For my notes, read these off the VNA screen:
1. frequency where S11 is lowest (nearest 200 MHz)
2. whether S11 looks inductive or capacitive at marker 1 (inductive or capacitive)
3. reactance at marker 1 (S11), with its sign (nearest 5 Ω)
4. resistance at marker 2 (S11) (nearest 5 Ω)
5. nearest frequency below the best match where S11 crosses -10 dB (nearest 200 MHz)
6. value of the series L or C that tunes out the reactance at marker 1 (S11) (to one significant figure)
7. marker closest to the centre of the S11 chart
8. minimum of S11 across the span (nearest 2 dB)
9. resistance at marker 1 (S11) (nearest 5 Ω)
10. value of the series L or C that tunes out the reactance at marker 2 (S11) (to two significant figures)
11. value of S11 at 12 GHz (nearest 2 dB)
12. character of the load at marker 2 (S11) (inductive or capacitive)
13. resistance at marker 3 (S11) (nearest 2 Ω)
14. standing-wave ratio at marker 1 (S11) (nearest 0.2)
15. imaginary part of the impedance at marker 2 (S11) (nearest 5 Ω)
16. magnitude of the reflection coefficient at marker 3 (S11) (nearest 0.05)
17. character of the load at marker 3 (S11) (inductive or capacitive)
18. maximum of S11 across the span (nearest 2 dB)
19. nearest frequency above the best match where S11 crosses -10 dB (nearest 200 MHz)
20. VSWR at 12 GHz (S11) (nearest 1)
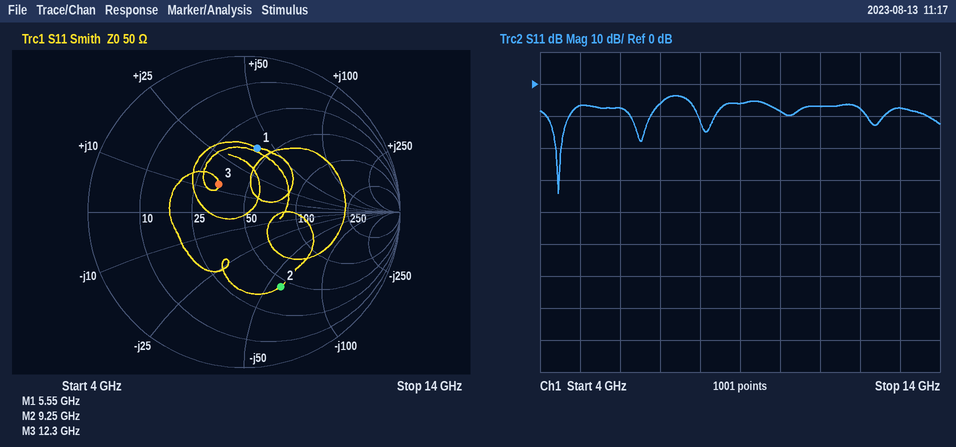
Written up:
4.4 GHz
inductive
+40 Ω
45 Ω
4.2 GHz
700 fF
marker 3
-34 dB
40 Ω
1.0 nH
-8 dB
capacitive
34 Ω
2.4
-60 Ω
0.25
inductive
-4 dB
4.8 GHz
2
